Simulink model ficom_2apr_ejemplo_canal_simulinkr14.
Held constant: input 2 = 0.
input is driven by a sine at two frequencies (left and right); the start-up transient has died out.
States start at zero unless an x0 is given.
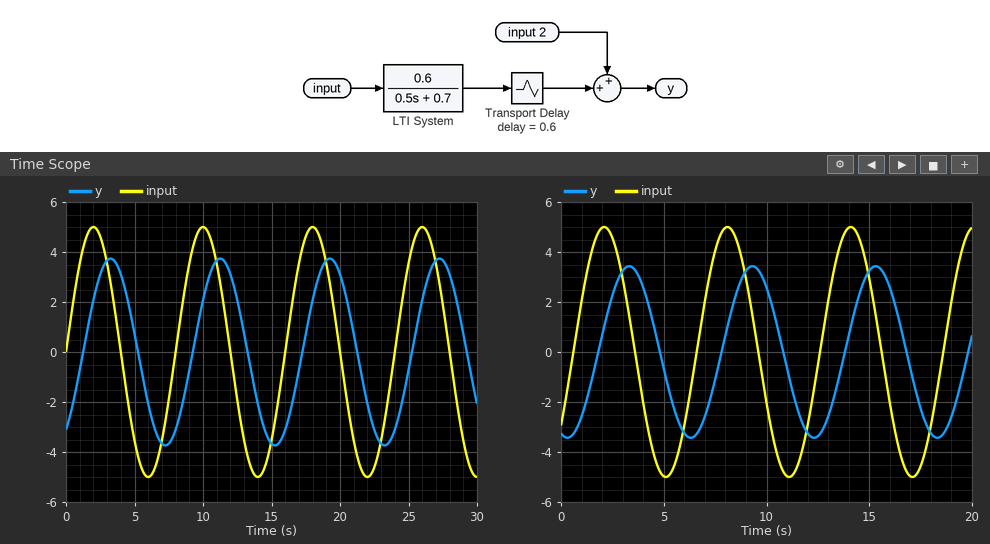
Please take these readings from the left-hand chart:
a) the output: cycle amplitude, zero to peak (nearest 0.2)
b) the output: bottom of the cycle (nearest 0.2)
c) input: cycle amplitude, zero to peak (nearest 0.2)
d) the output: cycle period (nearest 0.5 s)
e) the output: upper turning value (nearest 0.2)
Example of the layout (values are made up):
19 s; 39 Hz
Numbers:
3.8; -3.8; 5.0; 8.0 s; 3.8
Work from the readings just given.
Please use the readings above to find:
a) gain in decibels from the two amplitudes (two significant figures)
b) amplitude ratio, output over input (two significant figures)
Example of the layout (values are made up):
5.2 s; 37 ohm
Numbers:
-2.4 dB; 0.76
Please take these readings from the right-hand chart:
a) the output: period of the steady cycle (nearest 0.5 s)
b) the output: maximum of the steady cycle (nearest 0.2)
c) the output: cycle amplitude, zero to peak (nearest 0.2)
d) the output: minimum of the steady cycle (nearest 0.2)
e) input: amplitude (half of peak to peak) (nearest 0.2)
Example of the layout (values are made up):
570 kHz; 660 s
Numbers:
6.0 s; 3.4; 3.4; -3.4; 5.0
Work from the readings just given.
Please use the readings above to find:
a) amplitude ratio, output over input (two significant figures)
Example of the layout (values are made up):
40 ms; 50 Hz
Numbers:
0.68
